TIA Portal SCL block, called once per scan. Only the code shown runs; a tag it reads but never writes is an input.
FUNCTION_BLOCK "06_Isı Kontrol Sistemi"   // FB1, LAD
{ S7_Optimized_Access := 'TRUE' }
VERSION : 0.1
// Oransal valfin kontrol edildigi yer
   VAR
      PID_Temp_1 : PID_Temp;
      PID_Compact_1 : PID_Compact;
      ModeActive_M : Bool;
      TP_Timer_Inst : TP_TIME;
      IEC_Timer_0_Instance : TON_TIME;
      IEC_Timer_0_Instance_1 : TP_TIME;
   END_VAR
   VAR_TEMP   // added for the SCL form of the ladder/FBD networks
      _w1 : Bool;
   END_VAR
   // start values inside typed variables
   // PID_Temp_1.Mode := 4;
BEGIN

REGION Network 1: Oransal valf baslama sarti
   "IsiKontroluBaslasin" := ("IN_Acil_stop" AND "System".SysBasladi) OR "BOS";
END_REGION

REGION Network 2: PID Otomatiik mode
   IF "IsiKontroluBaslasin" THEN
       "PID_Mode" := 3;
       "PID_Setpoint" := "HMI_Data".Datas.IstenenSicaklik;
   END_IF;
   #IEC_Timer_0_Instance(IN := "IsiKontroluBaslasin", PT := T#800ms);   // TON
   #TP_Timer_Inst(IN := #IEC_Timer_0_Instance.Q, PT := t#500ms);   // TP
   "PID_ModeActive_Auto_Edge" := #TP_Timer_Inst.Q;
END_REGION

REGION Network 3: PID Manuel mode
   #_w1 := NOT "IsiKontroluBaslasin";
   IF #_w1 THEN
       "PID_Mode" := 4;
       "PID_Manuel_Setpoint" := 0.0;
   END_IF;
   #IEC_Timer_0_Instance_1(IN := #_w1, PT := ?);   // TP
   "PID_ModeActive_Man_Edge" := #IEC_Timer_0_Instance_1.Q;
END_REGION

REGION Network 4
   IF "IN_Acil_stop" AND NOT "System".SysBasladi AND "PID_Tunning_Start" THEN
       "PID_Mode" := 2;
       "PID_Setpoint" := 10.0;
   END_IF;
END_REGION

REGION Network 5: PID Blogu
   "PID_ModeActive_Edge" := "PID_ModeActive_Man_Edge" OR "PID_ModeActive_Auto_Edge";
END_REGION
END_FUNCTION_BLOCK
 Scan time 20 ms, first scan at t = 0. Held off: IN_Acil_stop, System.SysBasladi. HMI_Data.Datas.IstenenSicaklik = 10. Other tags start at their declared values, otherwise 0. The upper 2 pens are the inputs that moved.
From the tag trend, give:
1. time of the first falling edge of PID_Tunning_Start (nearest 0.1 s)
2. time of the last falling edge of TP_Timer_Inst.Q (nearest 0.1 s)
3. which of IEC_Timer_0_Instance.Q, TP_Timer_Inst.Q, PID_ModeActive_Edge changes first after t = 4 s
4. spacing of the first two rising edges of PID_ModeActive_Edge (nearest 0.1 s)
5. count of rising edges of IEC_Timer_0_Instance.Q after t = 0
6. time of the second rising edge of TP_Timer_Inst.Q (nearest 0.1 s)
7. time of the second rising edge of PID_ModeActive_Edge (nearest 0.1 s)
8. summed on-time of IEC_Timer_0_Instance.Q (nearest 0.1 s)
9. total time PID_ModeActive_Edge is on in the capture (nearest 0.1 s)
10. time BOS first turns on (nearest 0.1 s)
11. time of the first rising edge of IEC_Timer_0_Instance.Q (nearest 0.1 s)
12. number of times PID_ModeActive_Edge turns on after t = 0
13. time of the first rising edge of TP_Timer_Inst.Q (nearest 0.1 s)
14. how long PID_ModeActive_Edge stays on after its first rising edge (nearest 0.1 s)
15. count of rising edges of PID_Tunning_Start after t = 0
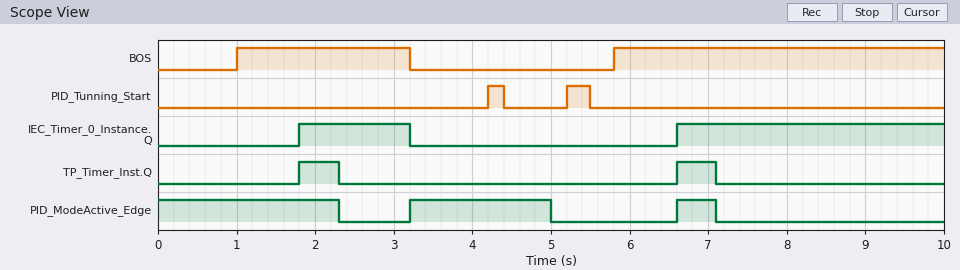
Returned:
4.4 s
7.1 s
PID_ModeActive_Edge
3.4 s
2
6.6 s
6.6 s
4.8 s
4.6 s
1.0 s
1.8 s
2
1.8 s
1.8 s
2
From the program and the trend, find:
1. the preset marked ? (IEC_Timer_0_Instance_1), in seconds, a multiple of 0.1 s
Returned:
1.8 s
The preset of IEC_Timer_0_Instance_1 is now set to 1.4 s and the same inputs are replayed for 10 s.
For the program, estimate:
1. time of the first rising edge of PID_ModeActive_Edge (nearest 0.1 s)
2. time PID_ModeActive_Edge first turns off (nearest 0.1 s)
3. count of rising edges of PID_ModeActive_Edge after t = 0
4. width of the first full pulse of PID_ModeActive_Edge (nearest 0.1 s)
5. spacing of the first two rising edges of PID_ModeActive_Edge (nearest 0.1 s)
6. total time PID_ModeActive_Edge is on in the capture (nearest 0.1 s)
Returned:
1.8 s
1.4 s
3
0.5 s
1.4 s
3.8 s
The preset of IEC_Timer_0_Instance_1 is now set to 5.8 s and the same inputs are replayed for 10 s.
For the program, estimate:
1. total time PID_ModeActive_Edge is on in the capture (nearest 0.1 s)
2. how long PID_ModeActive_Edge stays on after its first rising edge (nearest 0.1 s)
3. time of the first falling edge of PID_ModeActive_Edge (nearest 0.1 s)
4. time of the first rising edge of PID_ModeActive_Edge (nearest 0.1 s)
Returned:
6.3 s
0.5 s
5.8 s
6.6 s
